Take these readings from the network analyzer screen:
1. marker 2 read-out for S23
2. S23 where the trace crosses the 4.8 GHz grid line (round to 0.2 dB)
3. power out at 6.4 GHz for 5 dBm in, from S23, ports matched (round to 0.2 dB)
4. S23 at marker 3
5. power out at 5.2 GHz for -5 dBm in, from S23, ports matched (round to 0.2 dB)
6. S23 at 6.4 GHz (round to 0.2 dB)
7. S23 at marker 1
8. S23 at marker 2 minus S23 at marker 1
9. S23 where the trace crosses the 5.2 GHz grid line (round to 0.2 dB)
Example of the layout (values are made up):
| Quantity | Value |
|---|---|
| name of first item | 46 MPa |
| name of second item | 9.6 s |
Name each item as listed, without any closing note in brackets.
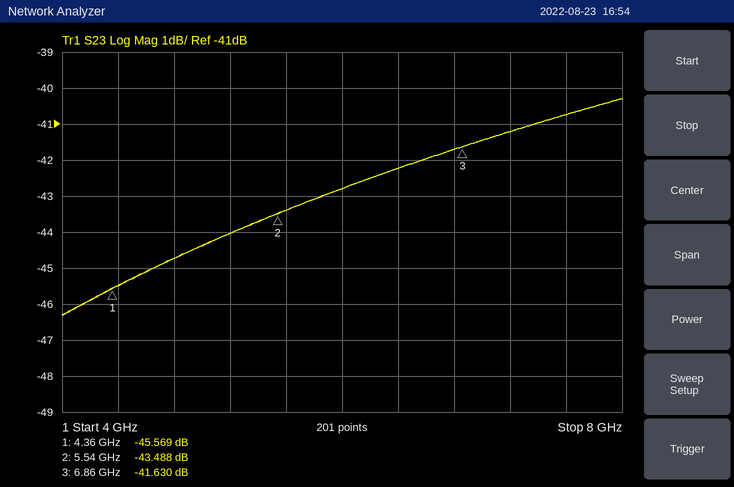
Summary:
| Quantity | Value |
|---|---|
| marker 2 read-out for S23 | -43.488 dB |
| S23 where the trace crosses the 4.8 GHz grid line | -44.8 dB |
| power out at 6.4 GHz for 5 dBm in, from S23, ports matched | -37.2 dBm |
| S23 at marker 3 | -41.630 dB |
| power out at 5.2 GHz for -5 dBm in, from S23, ports matched | -49.0 dBm |
| S23 at 6.4 GHz | -42.2 dB |
| S23 at marker 1 | -45.569 dB |
| S23 at marker 2 minus S23 at marker 1 | 2.081 dB |
| S23 where the trace crosses the 5.2 GHz grid line | -44.0 dB |
